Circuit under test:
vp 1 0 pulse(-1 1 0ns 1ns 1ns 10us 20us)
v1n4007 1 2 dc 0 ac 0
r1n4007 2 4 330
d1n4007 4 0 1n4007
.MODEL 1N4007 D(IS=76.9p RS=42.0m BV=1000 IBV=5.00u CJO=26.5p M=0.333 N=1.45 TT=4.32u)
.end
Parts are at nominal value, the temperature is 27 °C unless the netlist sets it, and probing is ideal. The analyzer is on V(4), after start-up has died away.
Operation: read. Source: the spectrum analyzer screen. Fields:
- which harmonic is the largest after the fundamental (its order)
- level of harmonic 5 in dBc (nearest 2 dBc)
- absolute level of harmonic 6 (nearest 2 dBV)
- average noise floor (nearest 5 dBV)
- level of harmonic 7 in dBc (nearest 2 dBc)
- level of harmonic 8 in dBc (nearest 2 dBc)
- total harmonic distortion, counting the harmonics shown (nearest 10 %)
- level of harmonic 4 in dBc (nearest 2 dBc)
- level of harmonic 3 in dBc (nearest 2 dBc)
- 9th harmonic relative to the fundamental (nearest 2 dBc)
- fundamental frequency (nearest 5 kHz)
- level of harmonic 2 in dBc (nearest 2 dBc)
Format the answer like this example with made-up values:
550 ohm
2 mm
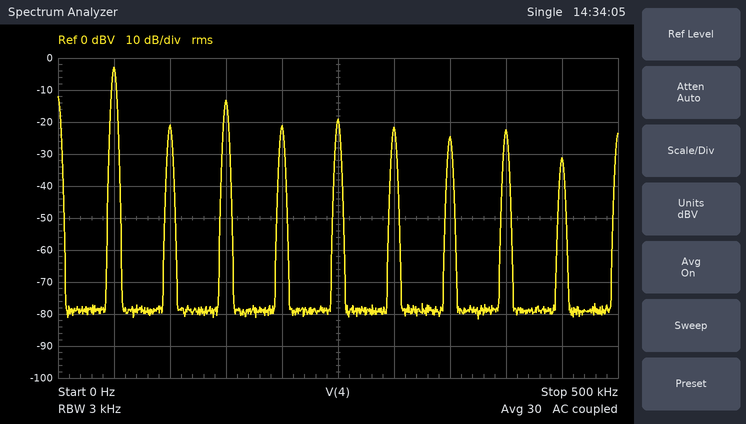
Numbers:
3
-16 dBc
-22 dBV
-80 dBV
-22 dBc
-20 dBc
40 %
-18 dBc
-10 dBc
-28 dBc
50 kHz
-18 dBc
